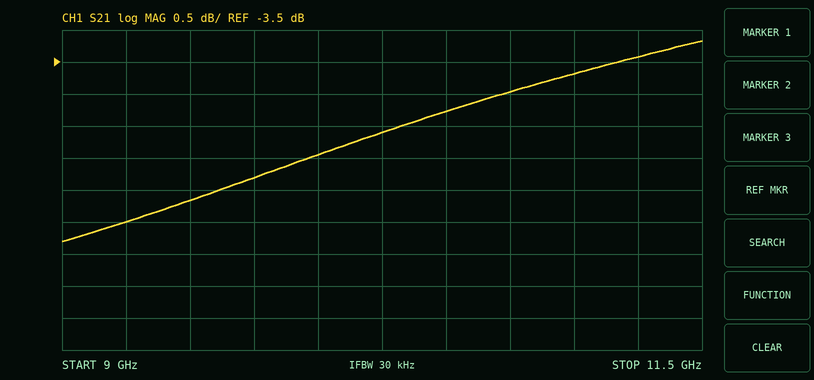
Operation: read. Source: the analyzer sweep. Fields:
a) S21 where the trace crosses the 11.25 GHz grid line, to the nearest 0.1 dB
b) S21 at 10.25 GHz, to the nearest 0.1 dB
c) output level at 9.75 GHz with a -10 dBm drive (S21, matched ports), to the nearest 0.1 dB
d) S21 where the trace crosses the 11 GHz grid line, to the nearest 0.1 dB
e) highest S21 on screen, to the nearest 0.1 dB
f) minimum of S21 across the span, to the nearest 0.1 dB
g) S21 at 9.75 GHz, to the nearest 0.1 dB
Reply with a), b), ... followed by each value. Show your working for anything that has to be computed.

a) -3.4 dB
b) -4.6 dB
c) -10 dBm + (-5.3 dB) = -15.3 dBm
d) -3.7 dB
e) -3.2 dB
f) -6.3 dB
g) -5.3 dB
